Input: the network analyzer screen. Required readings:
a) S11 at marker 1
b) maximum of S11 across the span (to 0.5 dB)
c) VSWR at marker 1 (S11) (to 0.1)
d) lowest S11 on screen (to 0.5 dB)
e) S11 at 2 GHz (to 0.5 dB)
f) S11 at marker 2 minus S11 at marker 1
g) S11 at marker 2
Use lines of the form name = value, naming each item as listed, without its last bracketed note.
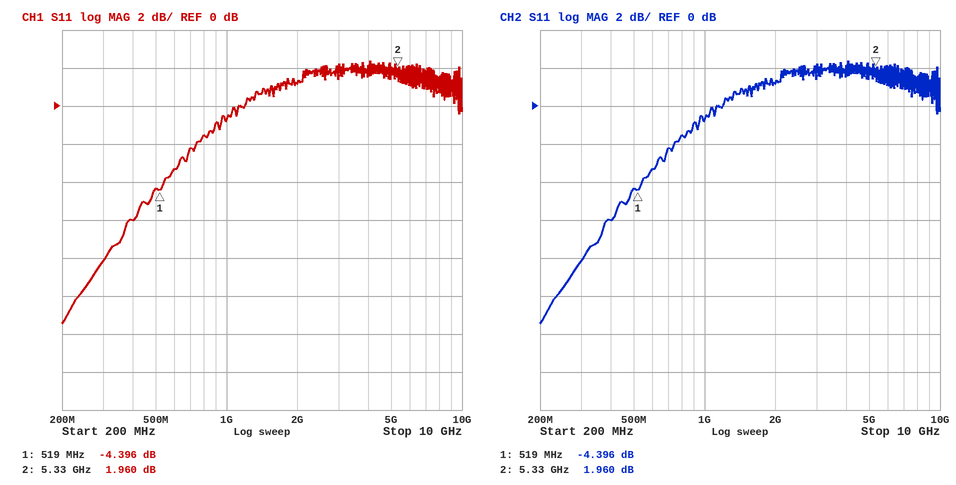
S11 at marker 1 = -4.396 dB
maximum of S11 across the span = 2.5 dB
VSWR at marker 1 (S11) = 4.0
lowest S11 on screen = -11.5 dB
S11 at 2 GHz = 1.0 dB
S11 at marker 2 minus S11 at marker 1 = 6.356 dB
S11 at marker 2 = 1.960 dB
